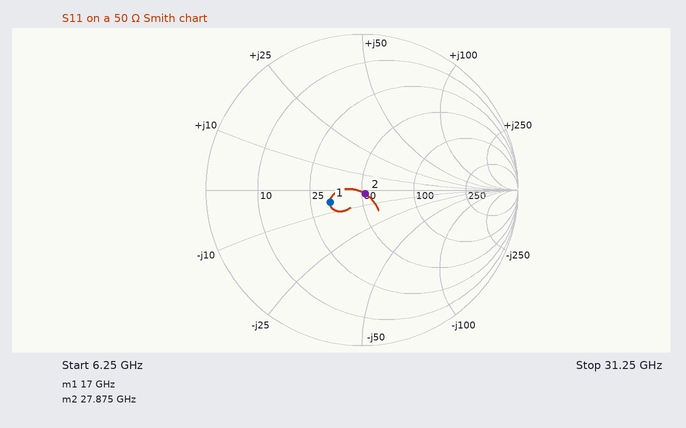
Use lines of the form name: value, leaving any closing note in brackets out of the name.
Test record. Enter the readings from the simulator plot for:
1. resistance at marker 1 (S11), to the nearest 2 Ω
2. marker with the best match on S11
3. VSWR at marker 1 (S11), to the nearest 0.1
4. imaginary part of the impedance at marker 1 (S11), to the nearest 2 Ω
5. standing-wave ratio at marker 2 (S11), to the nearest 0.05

resistance at marker 1 (S11), to the nearest 2 Ω: 32 Ω
marker with the best match on S11: marker 2
VSWR at marker 1 (S11), to the nearest 0.1: 1.6
imaginary part of the impedance at marker 1 (S11), to the nearest 2 Ω: -6 Ω
standing-wave ratio at marker 2 (S11), to the nearest 0.05: 1.05
